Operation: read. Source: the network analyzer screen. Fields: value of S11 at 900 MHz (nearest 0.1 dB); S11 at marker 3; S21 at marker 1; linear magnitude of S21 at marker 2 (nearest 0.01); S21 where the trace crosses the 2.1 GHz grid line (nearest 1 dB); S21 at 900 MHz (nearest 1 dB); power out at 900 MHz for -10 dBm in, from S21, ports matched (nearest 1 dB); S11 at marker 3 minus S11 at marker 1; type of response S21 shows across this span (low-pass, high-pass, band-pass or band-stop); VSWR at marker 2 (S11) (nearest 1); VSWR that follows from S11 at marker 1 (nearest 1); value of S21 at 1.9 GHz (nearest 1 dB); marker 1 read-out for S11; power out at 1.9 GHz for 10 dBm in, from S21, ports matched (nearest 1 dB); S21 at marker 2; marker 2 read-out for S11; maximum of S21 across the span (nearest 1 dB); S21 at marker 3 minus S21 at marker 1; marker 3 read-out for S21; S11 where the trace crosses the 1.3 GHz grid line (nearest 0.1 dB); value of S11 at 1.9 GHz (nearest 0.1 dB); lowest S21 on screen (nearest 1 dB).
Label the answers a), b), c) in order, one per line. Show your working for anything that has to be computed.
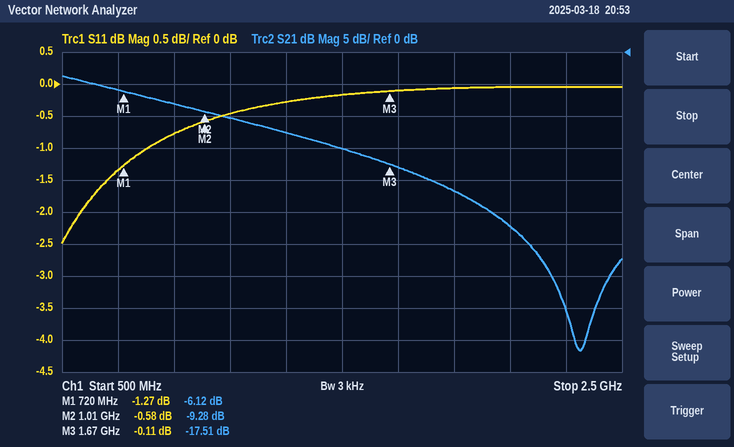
a) -0.8 dB
b) -0.11 dB
c) -6.12 dB
d) 10^(-9.28/20) ≈ 0.34
e) -27 dB
f) -8 dB
g) -10 dBm + (-8 dB) = -18 dBm
h) -0.11 − (-1.27) = 1.16 dB
i) low-pass
j) (1 + 0.9354)/(1 − 0.9354) ≈ 30
k) (1 + 0.8640)/(1 − 0.8640) ≈ 14
l) -22 dB
m) -1.27 dB
n) 10 dBm + (-22 dB) = -12 dBm
o) -9.28 dB
p) -0.58 dB
q) -4 dB
r) -17.51 − (-6.12) = -11.39 dB
s) -17.51 dB
t) -0.3 dB
u) -0.1 dB
v) -47 dB
